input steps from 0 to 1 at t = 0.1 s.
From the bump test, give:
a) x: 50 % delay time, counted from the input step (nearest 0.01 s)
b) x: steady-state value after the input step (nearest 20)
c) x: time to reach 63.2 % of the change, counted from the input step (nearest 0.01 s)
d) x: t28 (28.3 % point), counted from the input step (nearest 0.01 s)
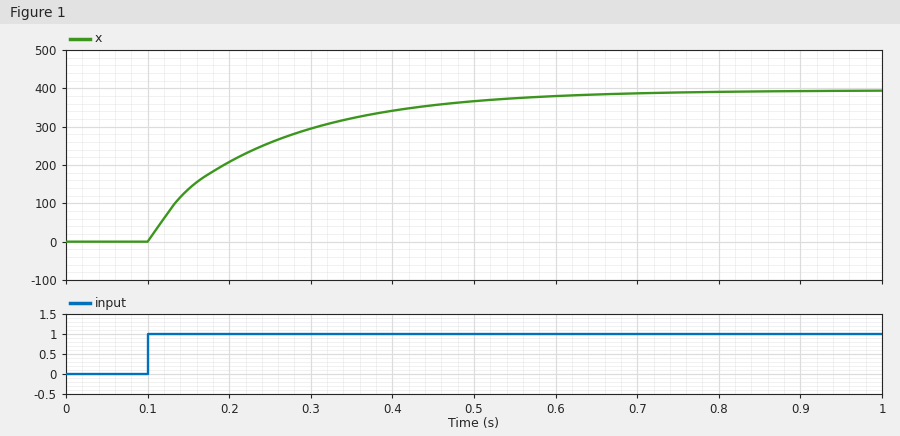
0.09 s
400
0.14 s
0.04 s
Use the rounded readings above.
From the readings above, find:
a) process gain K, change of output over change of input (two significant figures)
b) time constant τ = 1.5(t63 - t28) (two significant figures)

400
0.15 s
